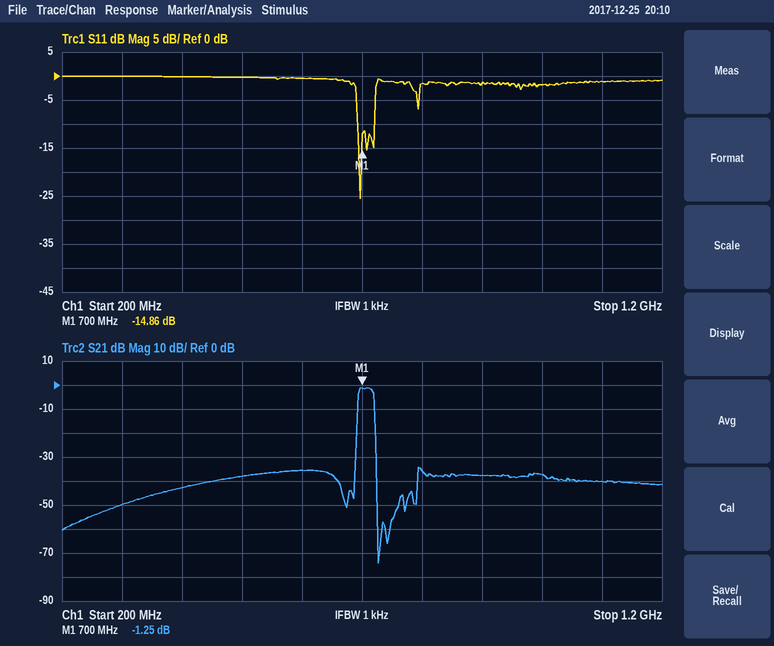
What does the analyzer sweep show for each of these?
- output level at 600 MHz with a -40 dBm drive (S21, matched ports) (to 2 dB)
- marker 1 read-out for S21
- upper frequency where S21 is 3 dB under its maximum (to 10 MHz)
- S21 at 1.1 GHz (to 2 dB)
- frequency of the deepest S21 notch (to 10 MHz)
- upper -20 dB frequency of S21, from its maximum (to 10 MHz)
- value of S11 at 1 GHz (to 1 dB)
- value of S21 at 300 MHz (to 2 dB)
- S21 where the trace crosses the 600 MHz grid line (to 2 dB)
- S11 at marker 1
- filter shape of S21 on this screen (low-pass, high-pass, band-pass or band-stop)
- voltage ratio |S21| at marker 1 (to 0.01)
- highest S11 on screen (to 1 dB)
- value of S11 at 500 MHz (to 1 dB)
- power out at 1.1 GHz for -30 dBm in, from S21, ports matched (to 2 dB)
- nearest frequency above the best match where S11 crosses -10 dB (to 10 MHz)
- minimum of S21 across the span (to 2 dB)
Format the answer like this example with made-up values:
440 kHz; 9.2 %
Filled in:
-76 dBm; -1.25 dB; 720 MHz; -40 dB; 730 MHz; 720 MHz; -2 dB; -50 dB; -36 dB; -14.86 dB; band-pass; 0.87; 0 dB; 0 dB; -70 dBm; 720 MHz; -74 dB
